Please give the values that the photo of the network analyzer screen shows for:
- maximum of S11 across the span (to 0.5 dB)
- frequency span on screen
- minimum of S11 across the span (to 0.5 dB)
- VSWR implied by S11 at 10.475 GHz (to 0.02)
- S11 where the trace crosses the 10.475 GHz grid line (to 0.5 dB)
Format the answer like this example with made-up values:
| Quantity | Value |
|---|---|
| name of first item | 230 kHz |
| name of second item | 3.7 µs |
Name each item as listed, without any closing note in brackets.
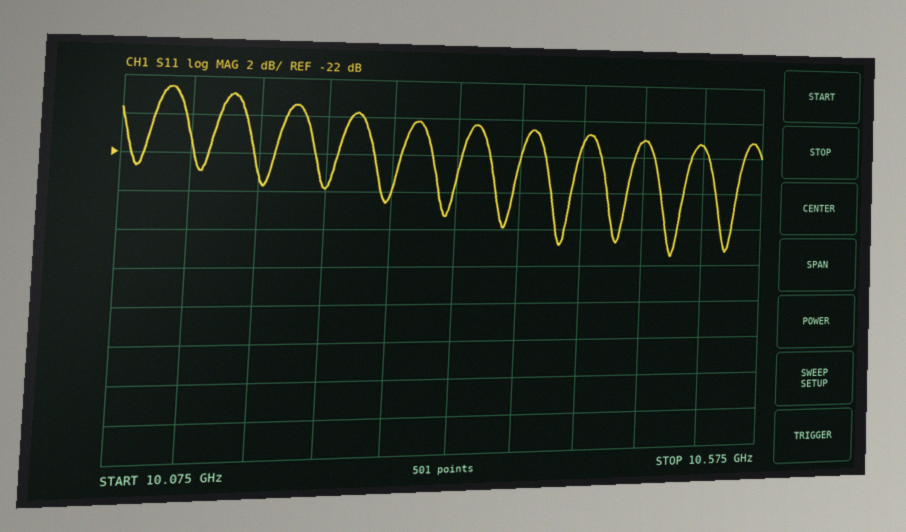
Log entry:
| Quantity | Value |
|---|---|
| maximum of S11 across the span | -18.5 dB |
| frequency span on screen | 500 MHz |
| minimum of S11 across the span | -27.5 dB |
| VSWR implied by S11 at 10.475 GHz | 1.20 |
| S11 where the trace crosses the 10.475 GHz grid line | -21.0 dB |
